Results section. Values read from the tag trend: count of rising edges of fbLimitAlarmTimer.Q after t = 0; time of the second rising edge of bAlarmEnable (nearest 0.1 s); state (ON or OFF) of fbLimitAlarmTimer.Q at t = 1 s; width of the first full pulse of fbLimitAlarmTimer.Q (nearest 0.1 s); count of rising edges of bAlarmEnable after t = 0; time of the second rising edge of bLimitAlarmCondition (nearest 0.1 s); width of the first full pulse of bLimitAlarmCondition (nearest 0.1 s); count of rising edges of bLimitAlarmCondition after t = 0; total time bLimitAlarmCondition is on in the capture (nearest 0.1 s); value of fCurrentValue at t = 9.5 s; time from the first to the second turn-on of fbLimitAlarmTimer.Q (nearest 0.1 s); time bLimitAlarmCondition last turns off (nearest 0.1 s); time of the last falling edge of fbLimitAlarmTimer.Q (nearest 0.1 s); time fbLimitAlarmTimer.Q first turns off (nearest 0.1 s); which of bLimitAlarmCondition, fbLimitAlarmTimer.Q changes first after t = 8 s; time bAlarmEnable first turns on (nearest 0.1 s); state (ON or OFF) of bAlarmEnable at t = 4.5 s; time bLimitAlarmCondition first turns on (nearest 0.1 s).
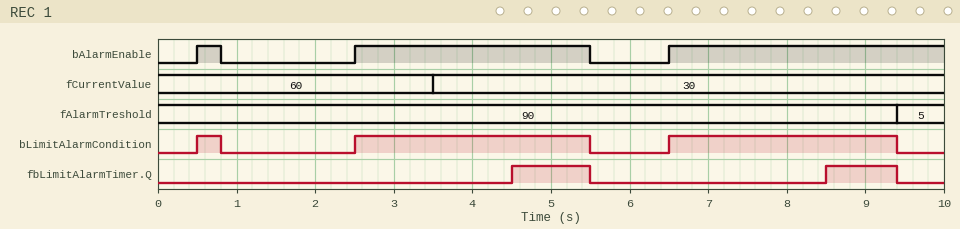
2
2.5 s
OFF
1.0 s
3
2.5 s
0.3 s
3
6.2 s
30
4.0 s
9.4 s
9.4 s
5.5 s
fbLimitAlarmTimer.Q
0.5 s
ON
0.5 s
